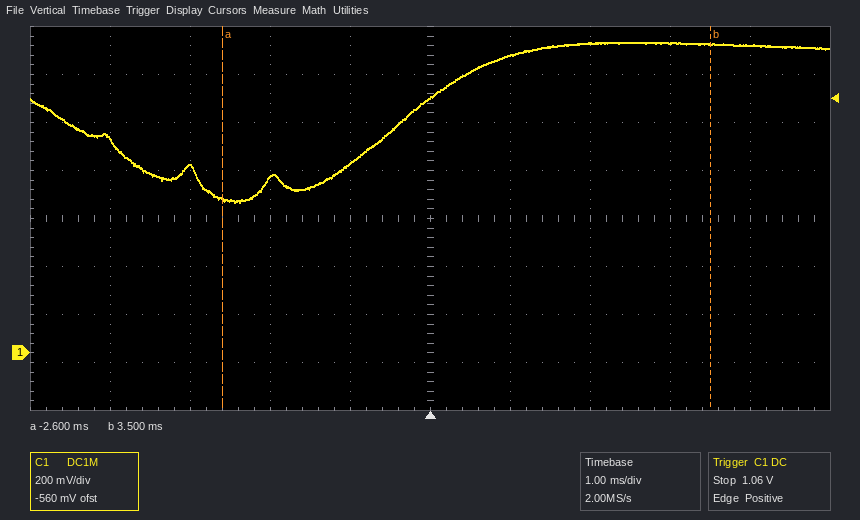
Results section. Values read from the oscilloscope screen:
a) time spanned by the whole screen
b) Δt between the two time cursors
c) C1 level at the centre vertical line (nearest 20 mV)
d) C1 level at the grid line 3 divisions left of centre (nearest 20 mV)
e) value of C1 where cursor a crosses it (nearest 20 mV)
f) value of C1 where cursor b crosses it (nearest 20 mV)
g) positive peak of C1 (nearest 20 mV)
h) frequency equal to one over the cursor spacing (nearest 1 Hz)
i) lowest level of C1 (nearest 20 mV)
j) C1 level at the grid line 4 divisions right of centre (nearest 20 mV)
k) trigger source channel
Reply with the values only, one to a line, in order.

10 ms
6.1 ms
1.06 V
780 mV
640 mV
1.28 V
1.30 V
164 Hz
620 mV
1.28 V
C1
